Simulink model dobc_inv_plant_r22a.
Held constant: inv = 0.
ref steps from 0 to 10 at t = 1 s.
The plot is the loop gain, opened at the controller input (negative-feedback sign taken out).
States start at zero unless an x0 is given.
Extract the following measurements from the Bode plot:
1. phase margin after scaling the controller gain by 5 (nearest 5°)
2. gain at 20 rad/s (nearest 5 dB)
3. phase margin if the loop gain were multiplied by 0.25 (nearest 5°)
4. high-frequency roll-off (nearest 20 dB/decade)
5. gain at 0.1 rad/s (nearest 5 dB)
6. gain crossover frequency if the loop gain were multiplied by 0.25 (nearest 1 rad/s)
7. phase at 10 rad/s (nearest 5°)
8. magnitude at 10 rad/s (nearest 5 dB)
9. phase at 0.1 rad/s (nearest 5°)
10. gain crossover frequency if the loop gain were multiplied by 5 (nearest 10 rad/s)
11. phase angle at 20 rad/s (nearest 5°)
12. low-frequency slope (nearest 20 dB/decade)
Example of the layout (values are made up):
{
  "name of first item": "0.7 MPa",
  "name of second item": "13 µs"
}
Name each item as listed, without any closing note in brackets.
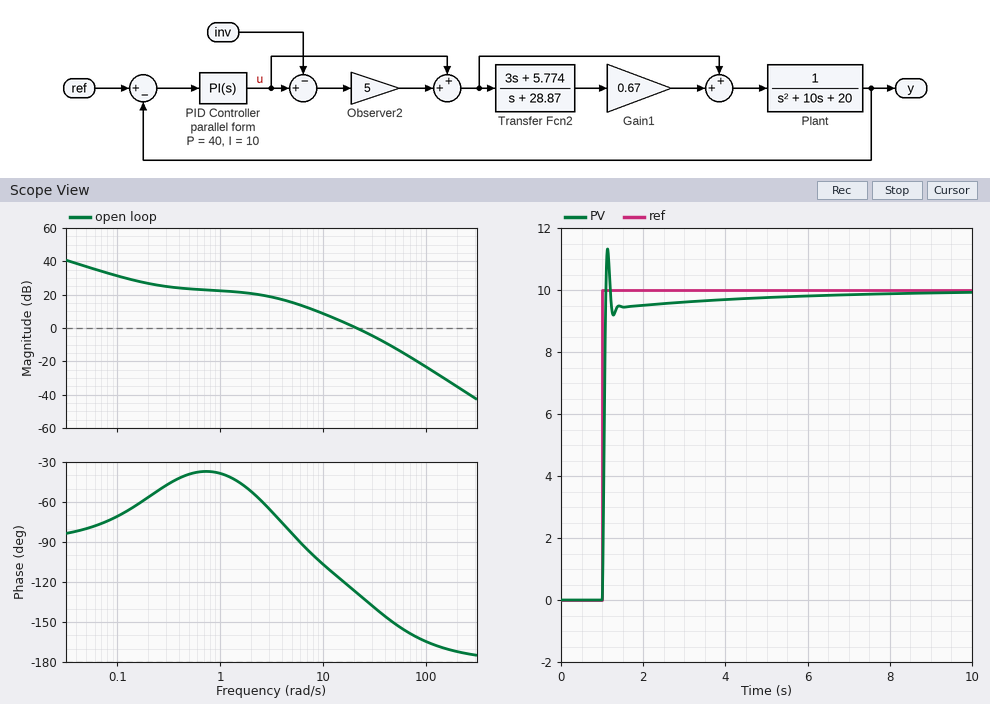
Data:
{
  "phase margin after scaling the controller gain by 5": "25°",
  "gain at 20 rad/s": "0 dB",
  "phase margin if the loop gain were multiplied by 0.25": "85°",
  "high-frequency roll-off": "-40 dB/decade",
  "gain at 0.1 rad/s": "30 dB",
  "gain crossover frequency if the loop gain were multiplied by 0.25": "7 rad/s",
  "phase at 10 rad/s": "-105°",
  "magnitude at 10 rad/s": "10 dB",
  "phase at 0.1 rad/s": "-70°",
  "gain crossover frequency if the loop gain were multiplied by 5": "60 rad/s",
  "phase angle at 20 rad/s": "-125°",
  "low-frequency slope": "-20 dB/decade"
}
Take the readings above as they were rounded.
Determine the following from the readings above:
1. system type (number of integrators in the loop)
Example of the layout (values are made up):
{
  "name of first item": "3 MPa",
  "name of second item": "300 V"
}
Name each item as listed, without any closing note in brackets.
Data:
{
  "system type": "1"
}
